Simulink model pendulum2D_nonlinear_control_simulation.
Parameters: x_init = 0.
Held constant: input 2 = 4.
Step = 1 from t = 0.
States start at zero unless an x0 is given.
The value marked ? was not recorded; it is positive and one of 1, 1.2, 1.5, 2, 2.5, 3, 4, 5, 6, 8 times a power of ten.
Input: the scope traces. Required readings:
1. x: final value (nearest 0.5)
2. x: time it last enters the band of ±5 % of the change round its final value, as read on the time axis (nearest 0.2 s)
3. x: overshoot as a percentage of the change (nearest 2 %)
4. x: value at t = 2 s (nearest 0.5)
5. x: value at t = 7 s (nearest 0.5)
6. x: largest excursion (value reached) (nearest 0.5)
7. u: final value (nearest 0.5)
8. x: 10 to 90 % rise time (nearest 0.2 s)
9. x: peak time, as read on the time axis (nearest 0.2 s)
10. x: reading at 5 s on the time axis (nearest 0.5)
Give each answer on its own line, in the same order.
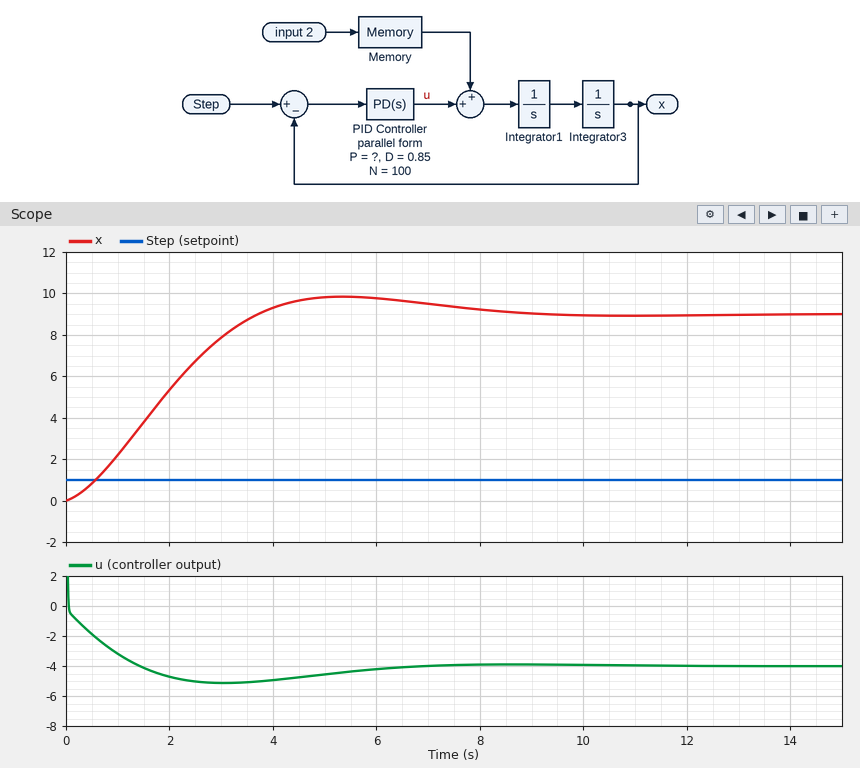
9.0
7.2 s
10 %
5.5
9.5
10.0
-4.0
2.6 s
5.4 s
10.0
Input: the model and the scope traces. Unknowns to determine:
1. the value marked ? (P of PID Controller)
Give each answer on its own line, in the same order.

0.5
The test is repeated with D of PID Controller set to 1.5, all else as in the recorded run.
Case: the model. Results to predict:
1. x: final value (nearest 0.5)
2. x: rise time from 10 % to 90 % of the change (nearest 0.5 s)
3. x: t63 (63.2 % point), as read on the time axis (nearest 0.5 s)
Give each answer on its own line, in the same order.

9.0
5.0 s
3.0 s
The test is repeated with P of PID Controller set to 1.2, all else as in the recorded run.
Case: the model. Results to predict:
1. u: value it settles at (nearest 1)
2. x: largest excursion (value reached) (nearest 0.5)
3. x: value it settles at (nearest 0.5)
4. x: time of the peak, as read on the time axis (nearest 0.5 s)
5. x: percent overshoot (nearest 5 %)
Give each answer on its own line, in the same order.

-4
5.5
4.5
3.0 s
25 %
